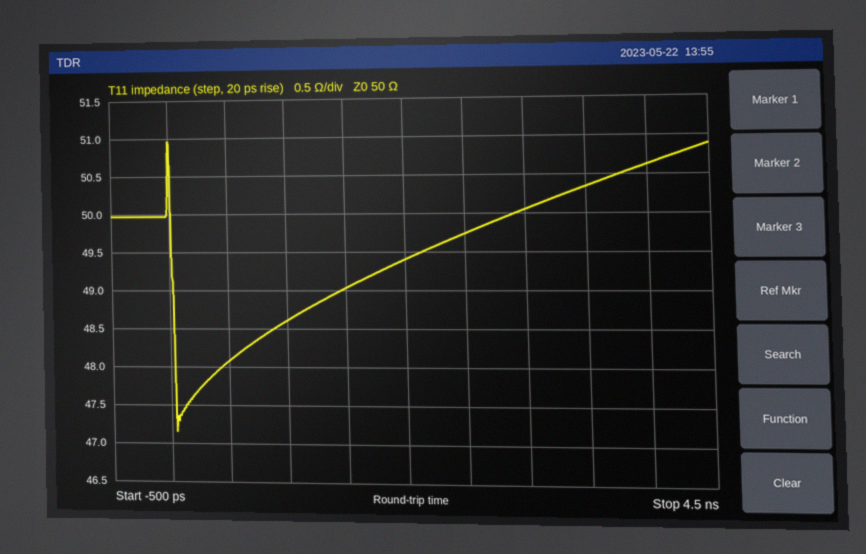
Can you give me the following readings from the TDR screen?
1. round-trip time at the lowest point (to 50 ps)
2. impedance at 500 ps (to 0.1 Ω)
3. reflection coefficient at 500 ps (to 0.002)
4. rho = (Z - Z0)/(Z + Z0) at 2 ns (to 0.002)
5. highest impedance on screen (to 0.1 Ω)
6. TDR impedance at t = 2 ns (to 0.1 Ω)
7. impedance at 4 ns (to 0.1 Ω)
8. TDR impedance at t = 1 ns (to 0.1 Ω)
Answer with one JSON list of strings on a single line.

["50 ps", "48.1 Ω", "-0.020", "-0.006", "51.0 Ω", "49.4 Ω", "50.6 Ω", "48.6 Ω"]
